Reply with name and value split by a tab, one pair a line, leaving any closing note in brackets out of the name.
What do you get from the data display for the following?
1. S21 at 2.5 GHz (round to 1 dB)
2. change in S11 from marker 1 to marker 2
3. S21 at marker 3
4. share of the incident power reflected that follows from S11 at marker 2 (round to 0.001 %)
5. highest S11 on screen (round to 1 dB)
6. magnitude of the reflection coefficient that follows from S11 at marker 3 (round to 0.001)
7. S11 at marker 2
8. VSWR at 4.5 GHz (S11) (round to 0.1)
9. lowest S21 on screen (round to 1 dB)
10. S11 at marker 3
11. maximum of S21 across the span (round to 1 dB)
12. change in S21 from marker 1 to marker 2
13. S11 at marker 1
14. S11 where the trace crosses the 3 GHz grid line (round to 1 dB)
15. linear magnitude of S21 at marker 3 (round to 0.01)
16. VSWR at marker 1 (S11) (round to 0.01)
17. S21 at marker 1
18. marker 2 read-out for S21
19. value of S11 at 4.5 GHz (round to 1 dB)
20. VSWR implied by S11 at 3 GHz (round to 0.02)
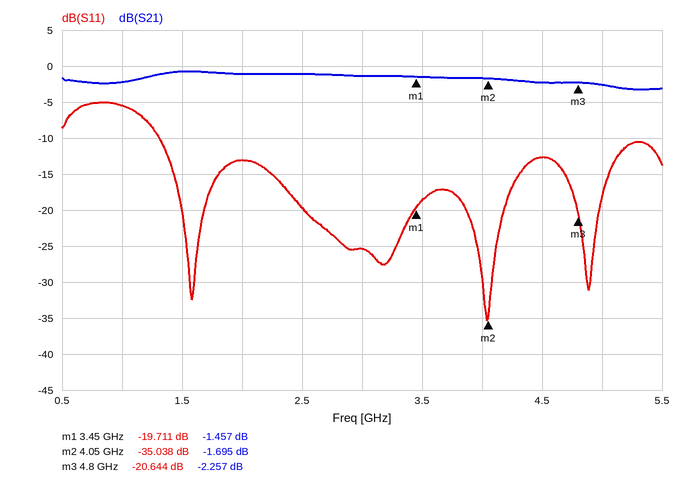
S21 at 2.5 GHz	-1 dB
change in S11 from marker 1 to marker 2	-15.327 dB
S21 at marker 3	-2.257 dB
share of the incident power reflected that follows from S11 at marker 2	0.031 %
highest S11 on screen	-5 dB
magnitude of the reflection coefficient that follows from S11 at marker 3	0.093
S11 at marker 2	-35.038 dB
VSWR at 4.5 GHz (S11)	1.6
lowest S21 on screen	-3 dB
S11 at marker 3	-20.644 dB
maximum of S21 across the span	-1 dB
change in S21 from marker 1 to marker 2	-0.238 dB
S11 at marker 1	-19.711 dB
S11 where the trace crosses the 3 GHz grid line	-25 dB
linear magnitude of S21 at marker 3	0.77
VSWR at marker 1 (S11)	1.23
S21 at marker 1	-1.457 dB
marker 2 read-out for S21	-1.695 dB
value of S11 at 4.5 GHz	-13 dB
VSWR implied by S11 at 3 GHz	1.12
